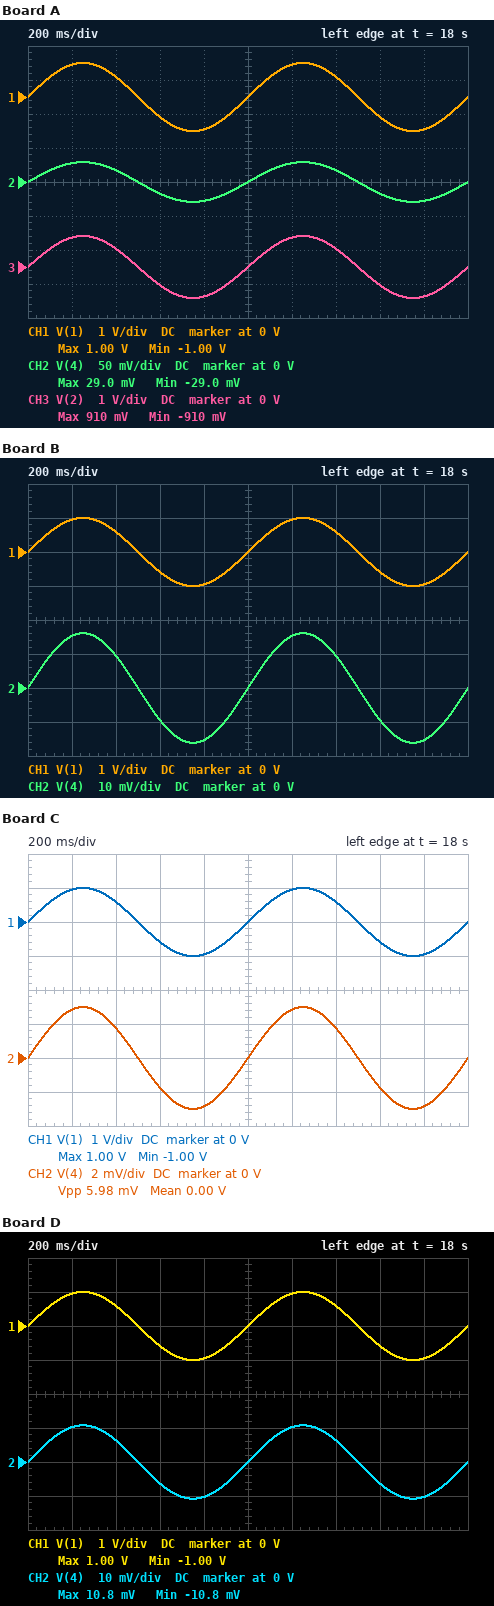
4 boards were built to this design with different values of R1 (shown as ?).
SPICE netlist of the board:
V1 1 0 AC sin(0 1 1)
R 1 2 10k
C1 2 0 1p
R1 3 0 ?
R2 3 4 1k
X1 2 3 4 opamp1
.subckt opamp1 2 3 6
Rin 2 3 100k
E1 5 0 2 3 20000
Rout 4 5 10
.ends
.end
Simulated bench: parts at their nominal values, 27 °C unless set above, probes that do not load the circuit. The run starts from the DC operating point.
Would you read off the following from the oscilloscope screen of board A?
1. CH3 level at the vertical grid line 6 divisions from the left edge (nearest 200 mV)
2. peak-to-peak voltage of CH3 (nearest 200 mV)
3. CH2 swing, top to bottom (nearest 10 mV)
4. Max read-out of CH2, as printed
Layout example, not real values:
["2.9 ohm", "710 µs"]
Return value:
["800 mV", "1.8 V", "60 mV", "29.0 mV"]
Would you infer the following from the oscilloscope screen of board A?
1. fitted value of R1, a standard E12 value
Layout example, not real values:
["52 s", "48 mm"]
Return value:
["3.3 kΩ"]
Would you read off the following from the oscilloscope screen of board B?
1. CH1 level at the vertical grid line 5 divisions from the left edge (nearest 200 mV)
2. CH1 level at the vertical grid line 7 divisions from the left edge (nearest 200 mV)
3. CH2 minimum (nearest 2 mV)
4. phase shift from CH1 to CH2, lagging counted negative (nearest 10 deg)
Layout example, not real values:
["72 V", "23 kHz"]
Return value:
["0 V", "600 mV", "-16 mV", "0 deg"]
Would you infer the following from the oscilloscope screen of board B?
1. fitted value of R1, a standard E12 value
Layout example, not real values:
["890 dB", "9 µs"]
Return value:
["1.8 kΩ"]
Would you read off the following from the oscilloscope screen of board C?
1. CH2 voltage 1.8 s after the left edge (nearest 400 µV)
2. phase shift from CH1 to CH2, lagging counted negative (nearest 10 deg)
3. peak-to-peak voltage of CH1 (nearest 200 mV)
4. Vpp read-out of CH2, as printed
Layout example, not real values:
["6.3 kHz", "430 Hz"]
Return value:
["-2.8 mV", "0 deg", "2.0 V", "5.98 mV"]
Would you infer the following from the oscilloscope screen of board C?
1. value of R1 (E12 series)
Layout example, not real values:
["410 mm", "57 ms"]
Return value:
["330 Ω"]
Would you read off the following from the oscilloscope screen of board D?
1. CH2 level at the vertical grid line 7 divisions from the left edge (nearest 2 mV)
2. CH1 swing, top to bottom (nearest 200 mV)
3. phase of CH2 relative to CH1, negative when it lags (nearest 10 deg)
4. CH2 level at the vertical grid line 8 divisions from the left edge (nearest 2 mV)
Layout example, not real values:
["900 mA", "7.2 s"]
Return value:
["6 mV", "2.0 V", "0 deg", "-6 mV"]
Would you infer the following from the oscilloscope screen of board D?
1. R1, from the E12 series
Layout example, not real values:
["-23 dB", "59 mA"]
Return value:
["1.2 kΩ"]
